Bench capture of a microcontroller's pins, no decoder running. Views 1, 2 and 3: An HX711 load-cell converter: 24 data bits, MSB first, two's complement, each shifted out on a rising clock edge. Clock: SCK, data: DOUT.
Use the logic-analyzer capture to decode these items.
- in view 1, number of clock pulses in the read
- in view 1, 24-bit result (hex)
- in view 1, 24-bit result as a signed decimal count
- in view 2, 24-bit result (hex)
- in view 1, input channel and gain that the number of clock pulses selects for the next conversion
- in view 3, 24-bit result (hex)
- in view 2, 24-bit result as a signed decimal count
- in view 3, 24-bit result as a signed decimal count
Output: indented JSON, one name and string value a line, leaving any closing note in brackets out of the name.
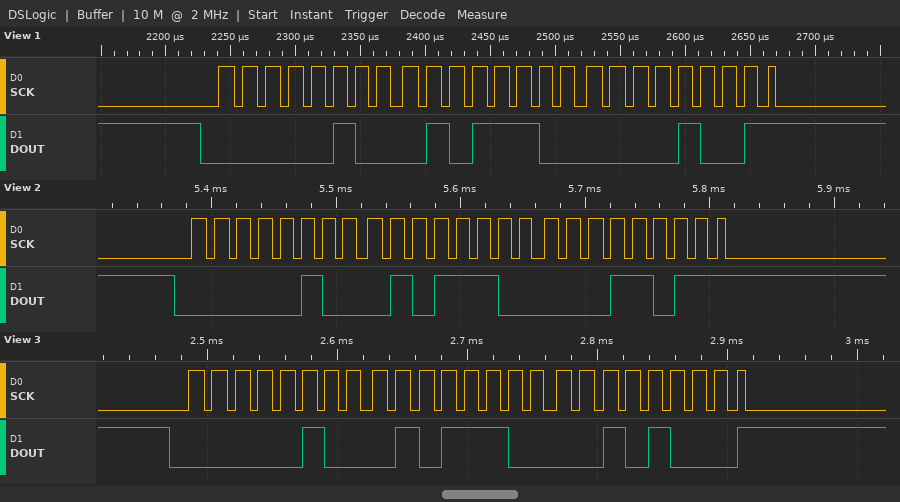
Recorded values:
{
  "in view 1, number of clock pulses in the read": "25",
  "in view 1, 24-bit result": "0x045C09",
  "in view 1, 24-bit result as a signed decimal count": "285705",
  "in view 2, 24-bit result": "0x045C1B",
  "in view 1, input channel and gain that the number of clock pulses selects for the next conversion": "channel A, gain 128",
  "in view 3, 24-bit result": "0x045C28",
  "in view 2, 24-bit result as a signed decimal count": "285723",
  "in view 3, 24-bit result as a signed decimal count": "285736"
}
